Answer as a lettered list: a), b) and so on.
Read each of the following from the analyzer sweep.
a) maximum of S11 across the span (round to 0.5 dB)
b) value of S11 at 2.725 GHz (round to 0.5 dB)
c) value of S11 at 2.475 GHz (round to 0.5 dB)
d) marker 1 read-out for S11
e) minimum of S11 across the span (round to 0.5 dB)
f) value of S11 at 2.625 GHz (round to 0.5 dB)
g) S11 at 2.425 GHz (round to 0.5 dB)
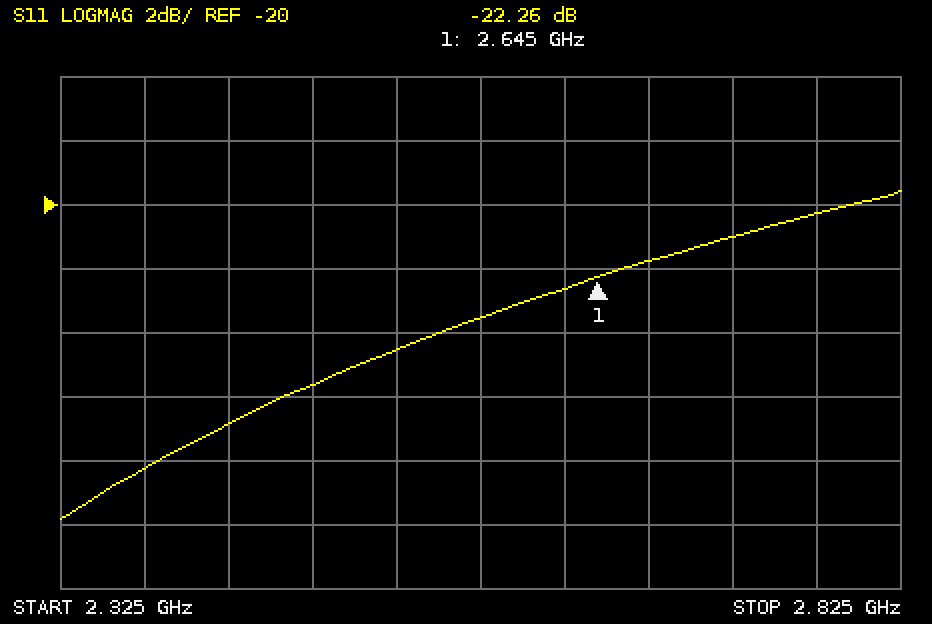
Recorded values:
a) -19.5 dB
b) -21.0 dB
c) -25.5 dB
d) -22.26 dB
e) -30.0 dB
f) -22.5 dB
g) -27.0 dB
